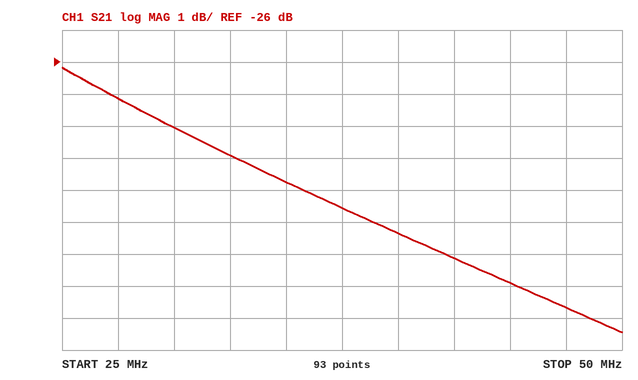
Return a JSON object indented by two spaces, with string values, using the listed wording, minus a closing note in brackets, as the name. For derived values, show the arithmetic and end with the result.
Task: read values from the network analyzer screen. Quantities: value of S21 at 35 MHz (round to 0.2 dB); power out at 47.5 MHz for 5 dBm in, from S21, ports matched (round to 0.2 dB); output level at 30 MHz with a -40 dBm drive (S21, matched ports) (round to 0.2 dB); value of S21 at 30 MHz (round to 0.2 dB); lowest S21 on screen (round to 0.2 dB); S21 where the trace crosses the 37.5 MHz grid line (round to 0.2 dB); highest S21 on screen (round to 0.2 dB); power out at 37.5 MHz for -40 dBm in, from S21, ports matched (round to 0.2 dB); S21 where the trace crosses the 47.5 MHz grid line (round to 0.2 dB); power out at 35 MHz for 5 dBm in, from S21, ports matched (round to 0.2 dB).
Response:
{
  "value of S21 at 35 MHz": "-29.8 dB",
  "power out at 47.5 MHz for 5 dBm in, from S21, ports matched": "5 dBm + (-33.6 dB) = -28.6 dBm",
  "output level at 30 MHz with a -40 dBm drive (S21, matched ports)": "-40 dBm + (-28.0 dB) = -68.0 dBm",
  "value of S21 at 30 MHz": "-28.0 dB",
  "lowest S21 on screen": "-34.4 dB",
  "S21 where the trace crosses the 37.5 MHz grid line": "-30.6 dB",
  "highest S21 on screen": "-26.2 dB",
  "power out at 37.5 MHz for -40 dBm in, from S21, ports matched": "-40 dBm + (-30.6 dB) = -70.6 dBm",
  "S21 where the trace crosses the 47.5 MHz grid line": "-33.6 dB",
  "power out at 35 MHz for 5 dBm in, from S21, ports matched": "5 dBm + (-29.8 dB) = -24.8 dBm"
}
